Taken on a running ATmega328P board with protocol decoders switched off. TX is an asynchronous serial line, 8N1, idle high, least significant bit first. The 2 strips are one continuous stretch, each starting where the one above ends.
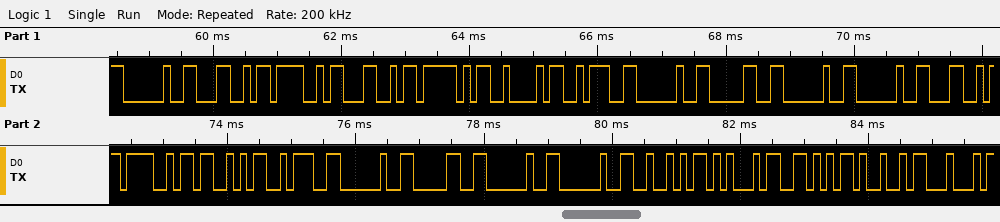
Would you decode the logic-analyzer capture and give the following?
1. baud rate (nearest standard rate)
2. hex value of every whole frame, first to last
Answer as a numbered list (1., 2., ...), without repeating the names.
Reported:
1. 9600 baud
2. 20 4C 4F 4C 5F 42 3A 20 30 20 20 4C 4F 53 3A 20 30 20 20 52 45 56 49 44
